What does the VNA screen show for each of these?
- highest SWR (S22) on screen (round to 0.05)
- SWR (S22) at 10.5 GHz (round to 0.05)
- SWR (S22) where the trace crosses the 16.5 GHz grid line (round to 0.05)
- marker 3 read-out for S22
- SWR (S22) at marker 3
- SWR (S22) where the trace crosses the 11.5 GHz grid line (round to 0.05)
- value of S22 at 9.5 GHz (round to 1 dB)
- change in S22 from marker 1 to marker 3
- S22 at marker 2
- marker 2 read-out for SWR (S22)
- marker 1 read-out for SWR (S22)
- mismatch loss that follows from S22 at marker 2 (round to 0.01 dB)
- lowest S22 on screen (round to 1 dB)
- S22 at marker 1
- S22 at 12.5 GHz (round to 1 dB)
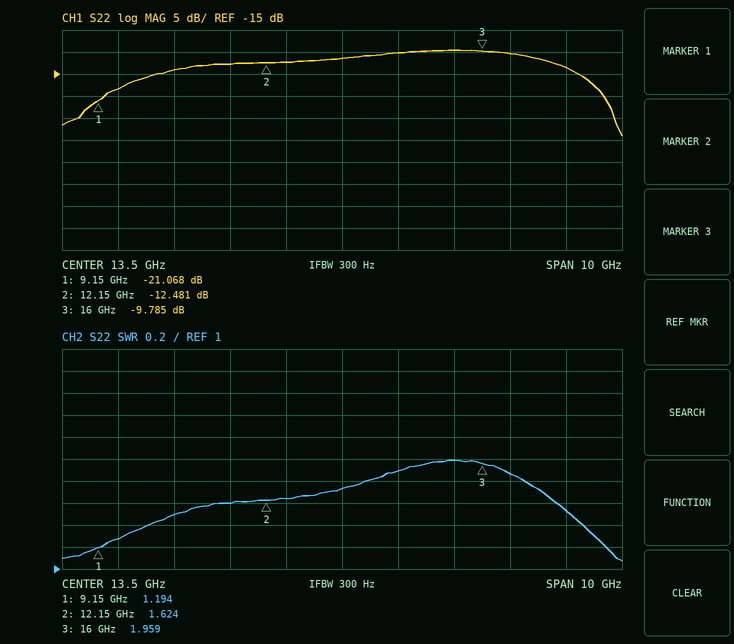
2.00
1.50
1.85
-9.785 dB
1.959
1.60
-18 dB
11.283 dB
-12.481 dB
1.624
1.194
0.25 dB
-29 dB
-21.068 dB
-12 dB
